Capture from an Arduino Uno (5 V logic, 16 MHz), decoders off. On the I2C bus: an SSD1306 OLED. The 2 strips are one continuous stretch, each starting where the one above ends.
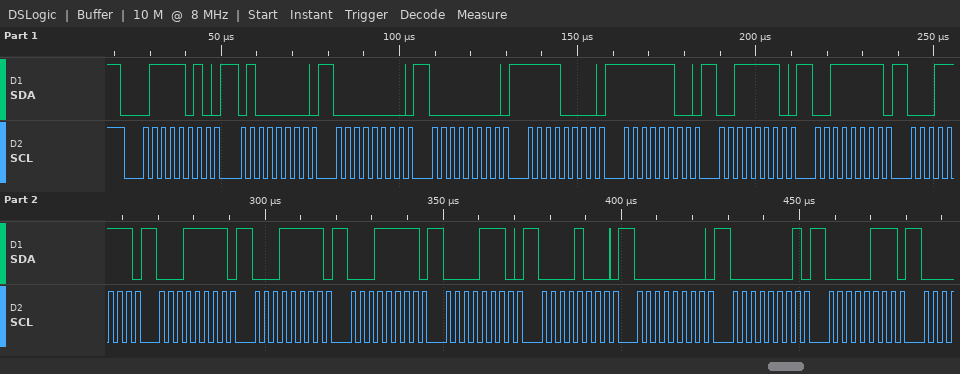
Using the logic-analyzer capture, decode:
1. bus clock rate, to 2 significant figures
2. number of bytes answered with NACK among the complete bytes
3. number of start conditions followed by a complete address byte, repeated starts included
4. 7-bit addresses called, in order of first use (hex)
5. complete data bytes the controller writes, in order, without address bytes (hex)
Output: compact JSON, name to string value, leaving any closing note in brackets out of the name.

{"bus clock rate, to 2 significant figures": "400 kHz", "number of bytes answered with NACK among the complete bytes": "0", "number of start conditions followed by a complete address byte, repeated starts included": "1", "7-bit addresses called, in order of first use": "0x3D", "complete data bytes the controller writes, in order, without address bytes": "40 00 00 F0 FC 3E 3F 1F 1F 1F 1F 0E 08 00 01 07"}
